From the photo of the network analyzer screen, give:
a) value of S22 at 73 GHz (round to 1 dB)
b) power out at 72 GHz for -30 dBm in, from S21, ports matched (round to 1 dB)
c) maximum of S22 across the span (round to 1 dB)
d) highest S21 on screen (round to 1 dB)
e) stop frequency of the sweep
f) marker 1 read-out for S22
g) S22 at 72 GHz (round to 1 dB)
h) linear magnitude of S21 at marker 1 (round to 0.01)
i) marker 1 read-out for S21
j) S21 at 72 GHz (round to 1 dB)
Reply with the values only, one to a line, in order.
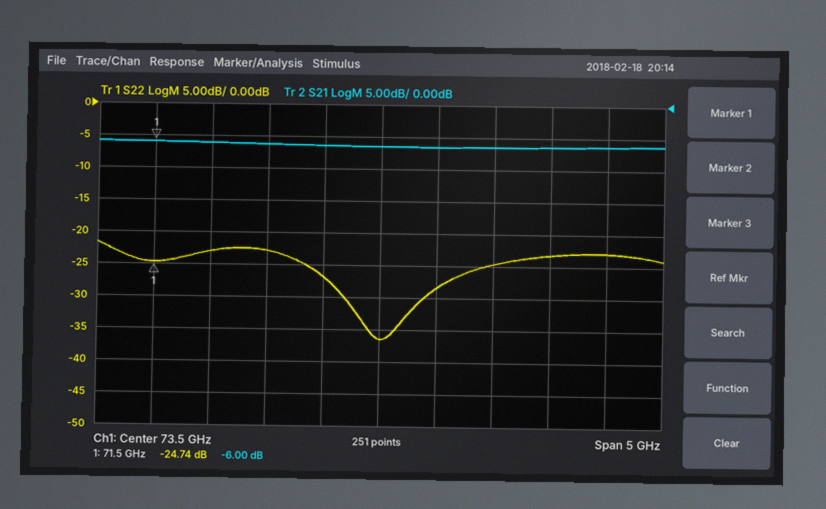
-27 dB
-36 dBm
-22 dB
-6 dB
76 GHz
-24.74 dB
-23 dB
0.50
-6.00 dB
-6 dB
